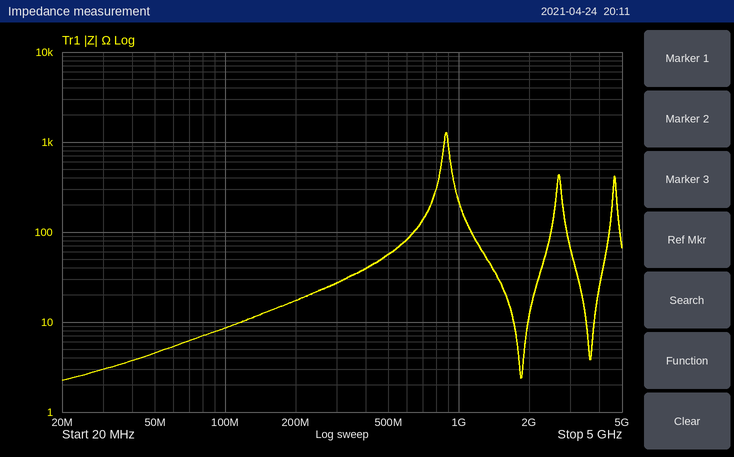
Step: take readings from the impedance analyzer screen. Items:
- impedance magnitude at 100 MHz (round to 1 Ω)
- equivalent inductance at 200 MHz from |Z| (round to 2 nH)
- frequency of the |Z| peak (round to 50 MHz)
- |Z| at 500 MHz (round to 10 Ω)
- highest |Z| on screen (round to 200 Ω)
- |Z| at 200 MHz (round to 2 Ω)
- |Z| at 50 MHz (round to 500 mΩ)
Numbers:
9 Ω
14 nH
900 MHz
60 Ω
1.2 kΩ
18 Ω
4.5 Ω
